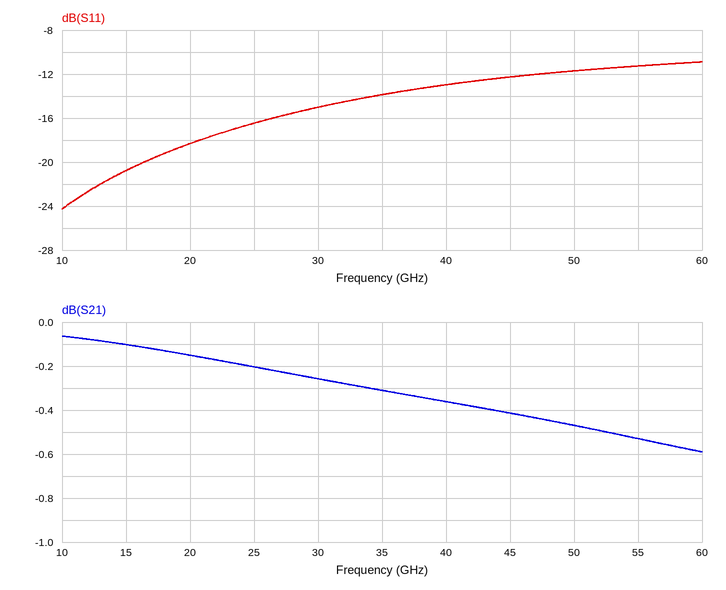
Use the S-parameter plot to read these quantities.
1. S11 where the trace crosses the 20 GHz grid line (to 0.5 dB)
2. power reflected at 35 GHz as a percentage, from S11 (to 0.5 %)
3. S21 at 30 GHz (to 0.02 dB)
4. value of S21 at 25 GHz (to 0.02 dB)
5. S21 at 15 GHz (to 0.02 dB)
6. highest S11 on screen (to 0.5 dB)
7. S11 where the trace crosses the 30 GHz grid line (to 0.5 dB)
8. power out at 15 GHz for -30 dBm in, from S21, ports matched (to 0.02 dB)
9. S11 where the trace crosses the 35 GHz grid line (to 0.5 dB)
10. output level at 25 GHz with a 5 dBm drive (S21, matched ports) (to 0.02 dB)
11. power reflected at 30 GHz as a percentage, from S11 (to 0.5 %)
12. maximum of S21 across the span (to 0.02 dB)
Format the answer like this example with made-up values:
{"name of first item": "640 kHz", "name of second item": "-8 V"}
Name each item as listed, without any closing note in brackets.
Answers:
{"S11 where the trace crosses the 20 GHz grid line": "-18.5 dB", "power reflected at 35 GHz as a percentage, from S11": "4.0 %", "S21 at 30 GHz": "-0.26 dB", "value of S21 at 25 GHz": "-0.20 dB", "S21 at 15 GHz": "-0.10 dB", "highest S11 on screen": "-11.0 dB", "S11 where the trace crosses the 30 GHz grid line": "-15.0 dB", "power out at 15 GHz for -30 dBm in, from S21, ports matched": "-30.10 dBm", "S11 where the trace crosses the 35 GHz grid line": "-14.0 dB", "output level at 25 GHz with a 5 dBm drive (S21, matched ports)": "4.80 dBm", "power reflected at 30 GHz as a percentage, from S11": "3.0 %", "maximum of S21 across the span": "-0.06 dB"}
